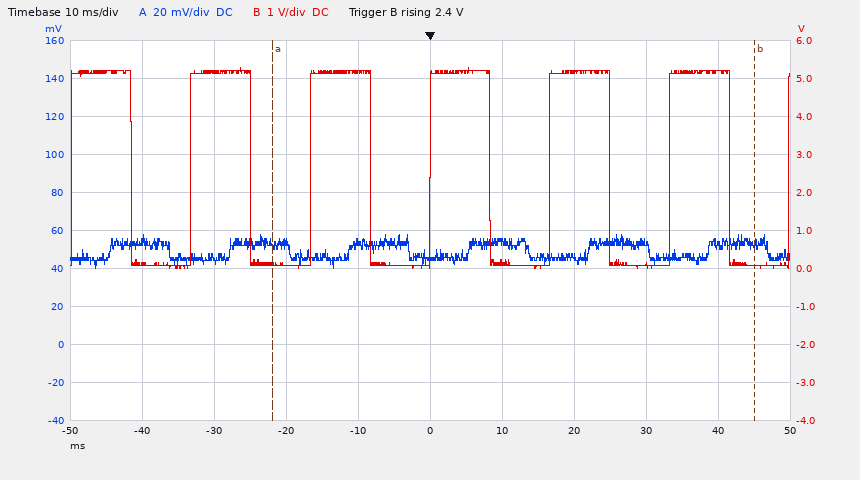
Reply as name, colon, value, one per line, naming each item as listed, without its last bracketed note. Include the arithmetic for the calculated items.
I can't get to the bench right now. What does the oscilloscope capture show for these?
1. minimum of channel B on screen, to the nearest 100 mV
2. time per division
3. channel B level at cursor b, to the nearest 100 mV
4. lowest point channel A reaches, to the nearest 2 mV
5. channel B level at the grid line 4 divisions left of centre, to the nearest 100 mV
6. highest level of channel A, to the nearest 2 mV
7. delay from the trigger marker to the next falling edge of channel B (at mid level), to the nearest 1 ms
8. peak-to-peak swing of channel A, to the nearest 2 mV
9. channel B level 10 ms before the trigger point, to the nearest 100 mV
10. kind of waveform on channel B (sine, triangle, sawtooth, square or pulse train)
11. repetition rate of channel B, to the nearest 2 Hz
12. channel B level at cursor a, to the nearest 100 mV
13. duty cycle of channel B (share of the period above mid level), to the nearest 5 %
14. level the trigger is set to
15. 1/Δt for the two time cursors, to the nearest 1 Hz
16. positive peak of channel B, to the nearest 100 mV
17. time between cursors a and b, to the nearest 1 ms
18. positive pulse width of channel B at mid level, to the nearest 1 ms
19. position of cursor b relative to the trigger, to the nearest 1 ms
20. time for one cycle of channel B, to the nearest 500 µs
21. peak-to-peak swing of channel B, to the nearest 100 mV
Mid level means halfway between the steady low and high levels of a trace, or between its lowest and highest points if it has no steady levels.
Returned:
minimum of channel B on screen, to the nearest 100 mV: 0.0 V
time per division: 10 ms
channel B level at cursor b, to the nearest 100 mV: 100 mV
lowest point channel A reaches, to the nearest 2 mV: 40 mV
channel B level at the grid line 4 divisions left of centre, to the nearest 100 mV: 100 mV
highest level of channel A, to the nearest 2 mV: 58 mV
delay from the trigger marker to the next falling edge of channel B (at mid level), to the nearest 1 ms: 8 ms
peak-to-peak swing of channel A, to the nearest 2 mV: 58 mV − (40 mV) = 18 mV
channel B level 10 ms before the trigger point, to the nearest 100 mV: 5.2 V
kind of waveform on channel B: square
repetition rate of channel B, to the nearest 2 Hz: 1 / 16.5 ms ≈ 60.6 Hz, so 60 Hz to the nearest 2 Hz
channel B level at cursor a, to the nearest 100 mV: 100 mV
duty cycle of channel B (share of the period above mid level), to the nearest 5 %: 8 ms / 16.5 ms ≈ 48.5 %, so 50 % to the nearest 5 %
level the trigger is set to: 2.4 V
1/Δt for the two time cursors, to the nearest 1 Hz: 1 / 67 ms ≈ 15 Hz
positive peak of channel B, to the nearest 100 mV: 5.3 V
time between cursors a and b, to the nearest 1 ms: 67 ms
positive pulse width of channel B at mid level, to the nearest 1 ms: 8 ms
position of cursor b relative to the trigger, to the nearest 1 ms: +45 ms
time for one cycle of channel B, to the nearest 500 µs: 16.5 ms
peak-to-peak swing of channel B, to the nearest 100 mV: 5.3 V − (0.0 V) = 5.3 V
